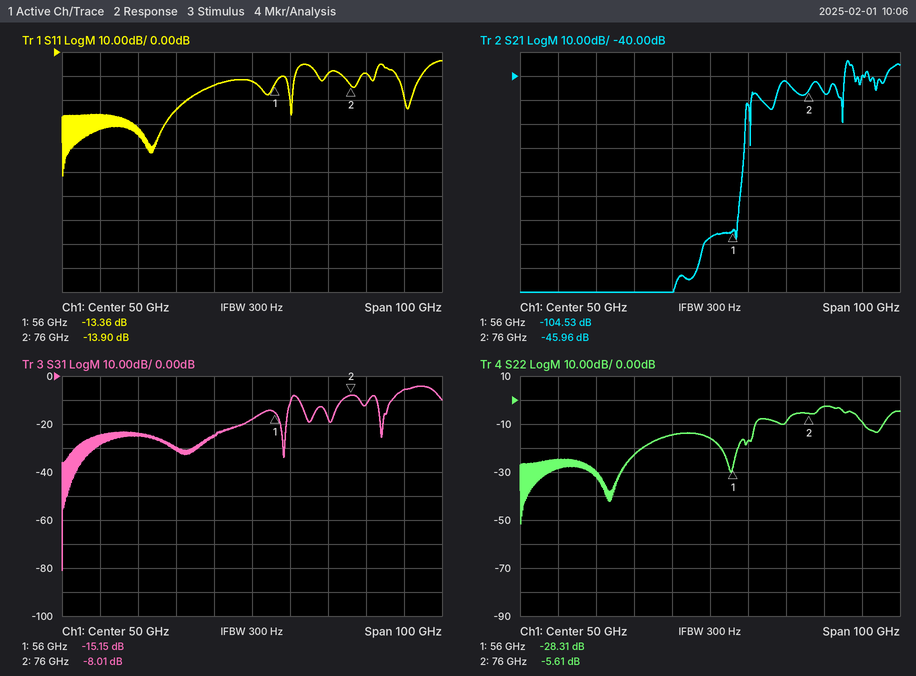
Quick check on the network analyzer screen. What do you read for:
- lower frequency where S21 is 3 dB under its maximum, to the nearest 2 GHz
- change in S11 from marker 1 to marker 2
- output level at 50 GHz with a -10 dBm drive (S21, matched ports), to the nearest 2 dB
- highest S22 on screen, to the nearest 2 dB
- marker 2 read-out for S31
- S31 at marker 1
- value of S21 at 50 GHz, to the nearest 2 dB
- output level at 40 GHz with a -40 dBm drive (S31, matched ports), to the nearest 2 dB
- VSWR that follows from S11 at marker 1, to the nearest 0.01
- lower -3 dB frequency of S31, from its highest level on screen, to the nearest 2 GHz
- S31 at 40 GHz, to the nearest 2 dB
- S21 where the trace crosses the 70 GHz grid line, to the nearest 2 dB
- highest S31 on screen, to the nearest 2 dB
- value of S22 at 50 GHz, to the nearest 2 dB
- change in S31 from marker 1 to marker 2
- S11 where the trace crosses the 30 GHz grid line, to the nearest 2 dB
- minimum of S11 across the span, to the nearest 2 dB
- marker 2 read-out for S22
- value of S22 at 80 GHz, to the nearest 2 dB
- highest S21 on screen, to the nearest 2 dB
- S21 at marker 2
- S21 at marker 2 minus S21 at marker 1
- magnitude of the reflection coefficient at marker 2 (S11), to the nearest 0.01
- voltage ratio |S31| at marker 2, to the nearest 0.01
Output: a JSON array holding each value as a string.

["86 GHz", "-0.54 dB", "-118 dBm", "-2 dB", "-8.01 dB", "-15.15 dB", "-108 dB", "-64 dBm", "1.55", "88 GHz", "-24 dB", "-42 dB", "-4 dB", "-16 dB", "7.14 dB", "-24 dB", "-52 dB", "-5.61 dB", "-2 dB", "-34 dB", "-45.96 dB", "58.57 dB", "0.20", "0.40"]
